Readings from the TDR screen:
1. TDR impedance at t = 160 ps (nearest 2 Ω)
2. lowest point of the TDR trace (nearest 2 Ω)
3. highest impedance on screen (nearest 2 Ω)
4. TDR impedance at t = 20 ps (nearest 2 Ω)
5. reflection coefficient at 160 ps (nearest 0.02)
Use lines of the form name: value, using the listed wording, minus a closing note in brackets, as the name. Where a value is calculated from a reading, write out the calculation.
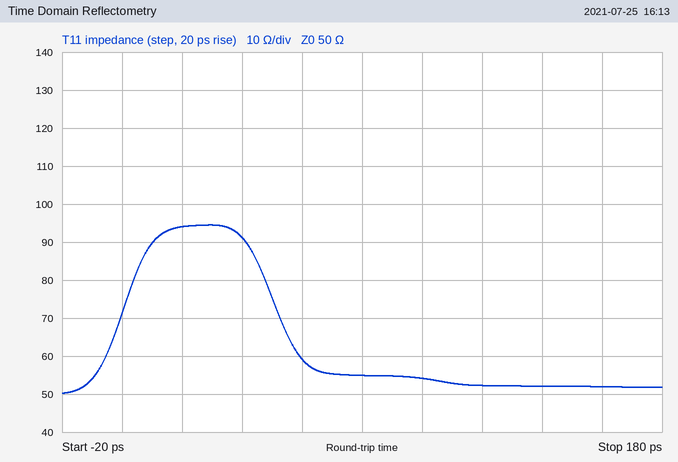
TDR impedance at t = 160 ps: 52 Ω
lowest point of the TDR trace: 50 Ω
highest impedance on screen: 94 Ω
TDR impedance at t = 20 ps: 94 Ω
reflection coefficient at 160 ps: (52 − 50)/(52 + 50) ≈ +0.02
